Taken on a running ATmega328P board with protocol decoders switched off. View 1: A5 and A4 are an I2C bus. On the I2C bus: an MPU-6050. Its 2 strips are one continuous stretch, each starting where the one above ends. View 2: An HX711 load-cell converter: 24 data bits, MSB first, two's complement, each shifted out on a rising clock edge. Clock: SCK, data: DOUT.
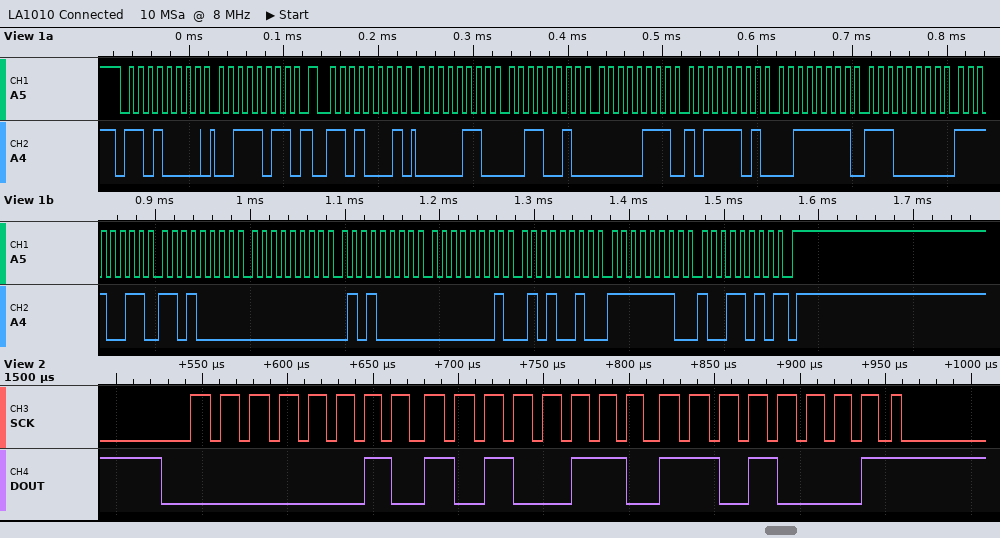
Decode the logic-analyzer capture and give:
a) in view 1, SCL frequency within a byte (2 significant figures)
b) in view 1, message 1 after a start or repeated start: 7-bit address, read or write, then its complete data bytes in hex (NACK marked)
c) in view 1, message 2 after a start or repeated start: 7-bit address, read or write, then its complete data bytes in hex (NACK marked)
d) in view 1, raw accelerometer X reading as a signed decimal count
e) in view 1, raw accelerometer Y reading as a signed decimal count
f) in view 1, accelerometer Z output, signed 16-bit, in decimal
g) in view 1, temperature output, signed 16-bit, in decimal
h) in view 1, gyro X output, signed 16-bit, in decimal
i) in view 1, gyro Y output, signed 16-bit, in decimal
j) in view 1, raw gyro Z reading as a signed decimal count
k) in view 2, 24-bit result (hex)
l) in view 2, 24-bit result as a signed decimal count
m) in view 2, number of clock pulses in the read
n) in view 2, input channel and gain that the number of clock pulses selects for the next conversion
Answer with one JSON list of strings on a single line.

["100 kHz", "0x68 write: 3B", "0x68 read: 06 32 07 BD 3F E0 F3 D0 00 50 01 52 FE 9A NACK", "1586", "1981", "16352", "-3120", "80", "338", "-358", "0x02A6D1", "173777", "25", "channel A, gain 128"]
